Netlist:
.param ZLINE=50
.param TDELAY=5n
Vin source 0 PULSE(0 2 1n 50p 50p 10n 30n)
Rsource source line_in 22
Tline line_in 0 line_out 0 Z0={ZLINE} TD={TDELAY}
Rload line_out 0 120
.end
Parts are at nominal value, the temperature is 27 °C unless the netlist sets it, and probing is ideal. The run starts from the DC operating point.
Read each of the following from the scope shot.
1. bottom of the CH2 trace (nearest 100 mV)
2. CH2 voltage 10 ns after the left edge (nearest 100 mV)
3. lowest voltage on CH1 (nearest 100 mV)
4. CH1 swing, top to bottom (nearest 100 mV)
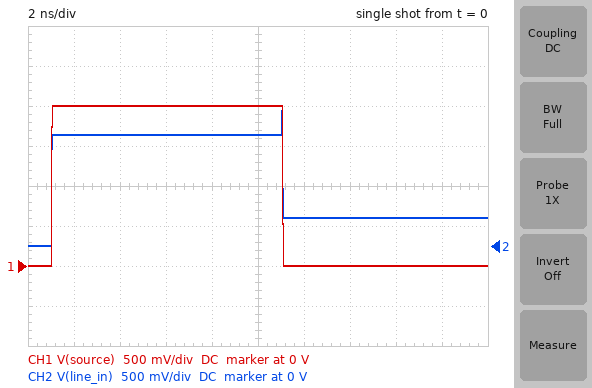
0 V
1.4 V
0 V
2.0 V
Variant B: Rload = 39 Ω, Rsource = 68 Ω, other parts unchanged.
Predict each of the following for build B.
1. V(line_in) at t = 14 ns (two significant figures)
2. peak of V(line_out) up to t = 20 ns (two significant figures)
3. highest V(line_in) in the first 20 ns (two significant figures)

-120 mV
740 mV
850 mV
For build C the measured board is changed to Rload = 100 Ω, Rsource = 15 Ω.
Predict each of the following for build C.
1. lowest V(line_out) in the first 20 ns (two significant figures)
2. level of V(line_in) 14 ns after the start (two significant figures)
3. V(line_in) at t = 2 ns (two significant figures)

-370 mV
240 mV
1.5 V
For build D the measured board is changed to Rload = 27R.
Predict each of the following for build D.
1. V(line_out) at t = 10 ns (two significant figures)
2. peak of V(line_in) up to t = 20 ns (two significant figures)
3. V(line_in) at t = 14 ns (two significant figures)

970 mV
1.4 V
-250 mV
